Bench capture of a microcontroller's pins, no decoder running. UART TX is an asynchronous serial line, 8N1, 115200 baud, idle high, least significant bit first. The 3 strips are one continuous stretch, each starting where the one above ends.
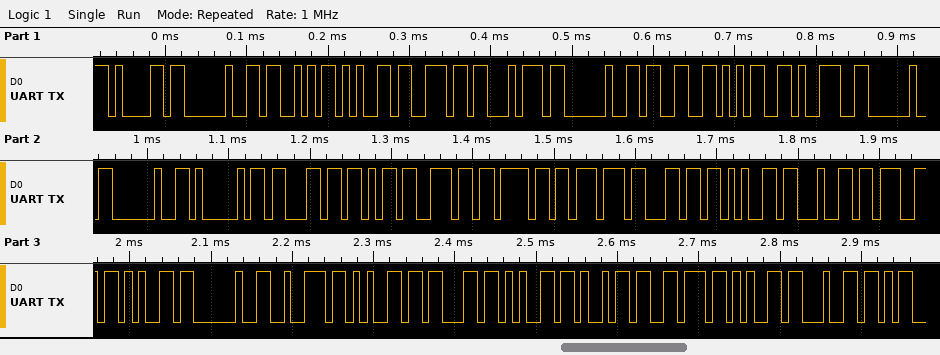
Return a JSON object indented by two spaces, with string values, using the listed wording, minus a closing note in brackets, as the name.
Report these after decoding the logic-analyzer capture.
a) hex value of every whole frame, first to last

{
  "hex value of every whole frame, first to last": "61 20 53 65 6E 74 20 33 35 39 20 20 41 63 6B 6E 6F 77 6C 65 64 67 65 20 72 65 63 65 69 76 65 64"
}
